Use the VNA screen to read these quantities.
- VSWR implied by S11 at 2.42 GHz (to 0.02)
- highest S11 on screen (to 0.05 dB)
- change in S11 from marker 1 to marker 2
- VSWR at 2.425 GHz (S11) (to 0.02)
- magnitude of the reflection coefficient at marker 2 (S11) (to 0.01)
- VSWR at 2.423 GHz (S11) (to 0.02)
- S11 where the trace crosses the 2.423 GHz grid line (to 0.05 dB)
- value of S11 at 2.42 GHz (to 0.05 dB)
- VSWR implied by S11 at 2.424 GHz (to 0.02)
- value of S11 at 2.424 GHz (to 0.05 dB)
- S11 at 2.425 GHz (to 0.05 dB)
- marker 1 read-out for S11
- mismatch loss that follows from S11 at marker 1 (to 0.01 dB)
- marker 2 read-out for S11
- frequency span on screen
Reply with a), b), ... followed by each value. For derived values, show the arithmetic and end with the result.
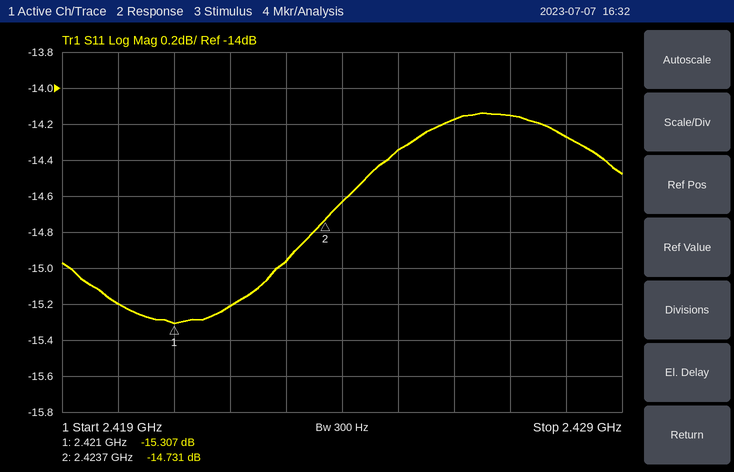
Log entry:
a) |Γ| = 10^(-15.2/20) = 0.1738; VSWR = (1 + 0.1738)/(1 − 0.1738) ≈ 1.42
b) -14.15 dB
c) -14.731 − (-15.307) = 0.576 dB
d) |Γ| = 10^(-14.35/20) = 0.1916; VSWR = (1 + 0.1916)/(1 − 0.1916) ≈ 1.47, so 1.48 to the nearest 0.02
e) 10^(-14.731/20) ≈ 0.18
f) |Γ| = 10^(-14.95/20) = 0.1789; VSWR = (1 + 0.1789)/(1 − 0.1789) ≈ 1.44
g) -14.95 dB
h) -15.20 dB
i) |Γ| = 10^(-14.65/20) = 0.1851; VSWR = (1 + 0.1851)/(1 − 0.1851) ≈ 1.45, so 1.46 to the nearest 0.02
j) -14.65 dB
k) -14.35 dB
l) -15.307 dB
m) −10 log10(1 − 10^(-15.307/10)) ≈ 0.13 dB
n) -14.731 dB
o) 10 MHz
